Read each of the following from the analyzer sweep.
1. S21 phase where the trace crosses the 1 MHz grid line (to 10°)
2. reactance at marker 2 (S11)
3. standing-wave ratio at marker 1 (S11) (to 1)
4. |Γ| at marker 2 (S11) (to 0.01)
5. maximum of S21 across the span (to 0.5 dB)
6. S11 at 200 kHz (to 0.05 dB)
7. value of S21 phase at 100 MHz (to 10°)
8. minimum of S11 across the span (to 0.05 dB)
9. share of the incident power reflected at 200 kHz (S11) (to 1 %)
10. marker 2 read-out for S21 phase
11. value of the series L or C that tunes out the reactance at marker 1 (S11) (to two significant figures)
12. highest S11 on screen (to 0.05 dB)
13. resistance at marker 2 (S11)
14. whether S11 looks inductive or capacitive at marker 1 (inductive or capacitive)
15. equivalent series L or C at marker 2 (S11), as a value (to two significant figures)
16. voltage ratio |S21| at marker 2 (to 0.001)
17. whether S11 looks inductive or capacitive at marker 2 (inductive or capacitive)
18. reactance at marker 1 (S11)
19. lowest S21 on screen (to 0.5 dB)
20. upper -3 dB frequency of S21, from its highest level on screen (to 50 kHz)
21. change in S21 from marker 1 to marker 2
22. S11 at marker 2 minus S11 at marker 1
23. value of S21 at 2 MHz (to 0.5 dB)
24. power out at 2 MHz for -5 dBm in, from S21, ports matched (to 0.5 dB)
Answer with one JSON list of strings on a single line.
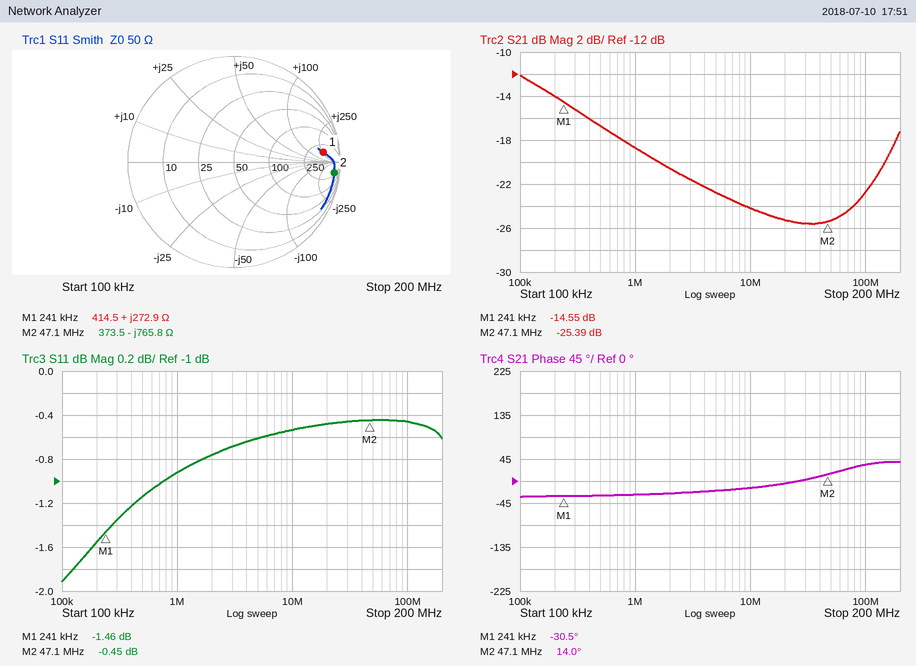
["-30°", "-765.8 Ω", "12", "0.95", "-12.0 dB", "-1.55 dB", "30°", "-1.90 dB", "70 %", "14.0°", "2.4 nF", "-0.45 dB", "373.5 Ω", "inductive", "4.4 pF", "0.054", "capacitive", "+272.9 Ω", "-25.5 dB", "300 kHz", "-10.84 dB", "1.01 dB", "-20.5 dB", "-25.5 dBm"]
